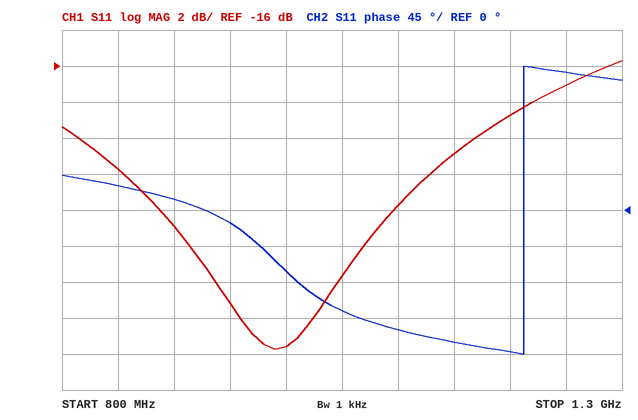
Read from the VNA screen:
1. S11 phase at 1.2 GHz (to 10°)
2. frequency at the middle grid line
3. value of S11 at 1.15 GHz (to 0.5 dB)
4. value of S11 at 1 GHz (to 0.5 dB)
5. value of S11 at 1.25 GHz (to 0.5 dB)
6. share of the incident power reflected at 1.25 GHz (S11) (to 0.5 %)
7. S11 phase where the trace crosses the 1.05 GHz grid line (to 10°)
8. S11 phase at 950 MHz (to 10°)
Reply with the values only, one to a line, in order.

-180°
1.05 GHz
-21.0 dB
-31.5 dB
-17.0 dB
2.0 %
-130°
-20°
